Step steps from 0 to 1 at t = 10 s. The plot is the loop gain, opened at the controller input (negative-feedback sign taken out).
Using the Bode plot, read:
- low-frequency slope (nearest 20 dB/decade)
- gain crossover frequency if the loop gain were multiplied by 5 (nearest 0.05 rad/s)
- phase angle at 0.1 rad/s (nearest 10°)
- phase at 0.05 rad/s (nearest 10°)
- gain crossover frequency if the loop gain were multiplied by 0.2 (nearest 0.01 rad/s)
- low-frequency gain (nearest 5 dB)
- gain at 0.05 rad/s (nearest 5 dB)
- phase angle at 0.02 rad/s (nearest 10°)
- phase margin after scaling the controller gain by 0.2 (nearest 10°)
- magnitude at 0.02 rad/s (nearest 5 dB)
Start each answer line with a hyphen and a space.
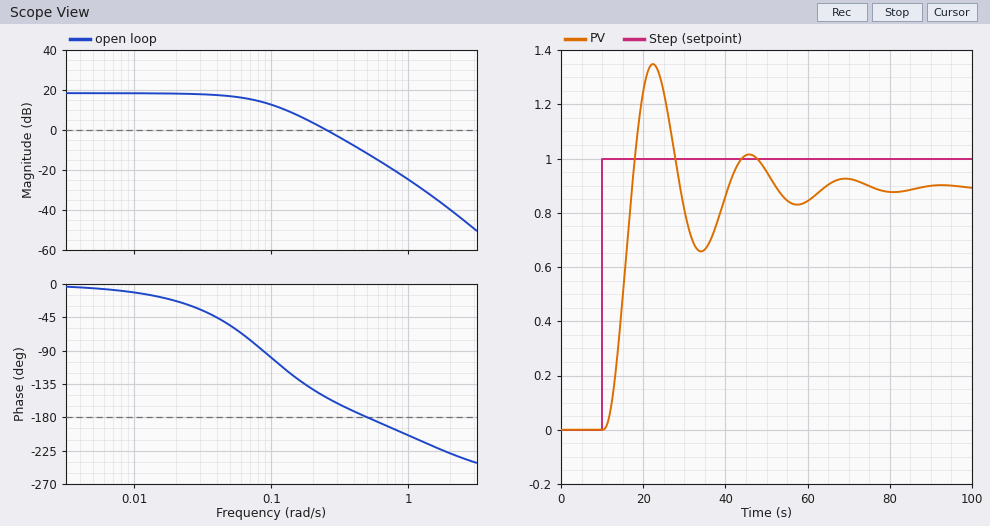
- 0 dB/decade
- 0.55 rad/s
- -100°
- -60°
- 0.09 rad/s
- 20 dB
- 15 dB
- -20°
- 90°
- 20 dB
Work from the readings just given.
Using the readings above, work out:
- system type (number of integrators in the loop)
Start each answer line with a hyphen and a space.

- 0
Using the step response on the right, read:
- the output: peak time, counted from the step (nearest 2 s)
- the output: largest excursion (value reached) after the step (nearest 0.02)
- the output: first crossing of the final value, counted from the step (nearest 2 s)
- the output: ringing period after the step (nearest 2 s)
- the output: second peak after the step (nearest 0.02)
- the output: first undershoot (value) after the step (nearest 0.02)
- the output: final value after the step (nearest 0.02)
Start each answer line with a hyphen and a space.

- 12 s
- 1.34
- 8 s
- 24 s
- 1.02
- 0.66
- 0.90
